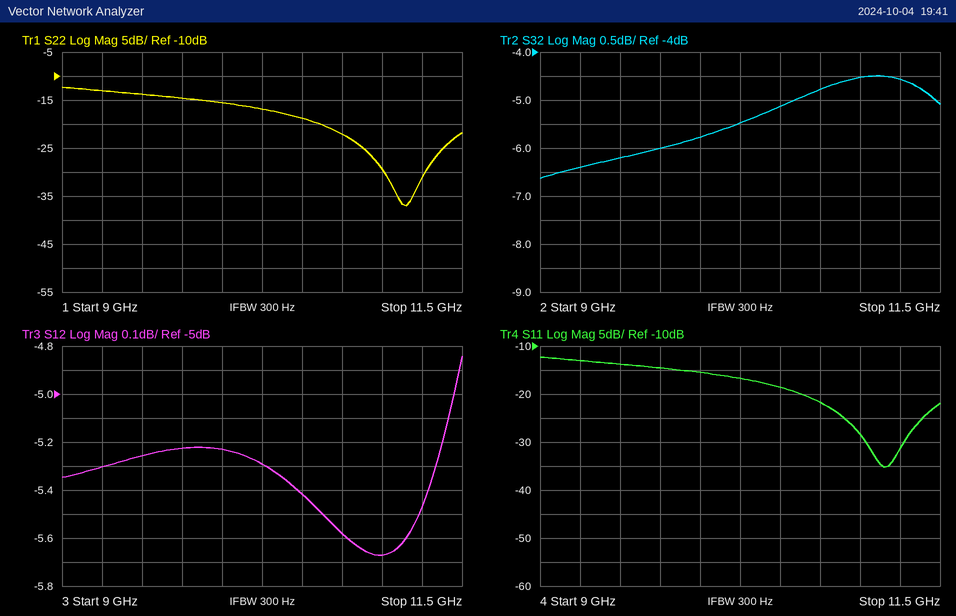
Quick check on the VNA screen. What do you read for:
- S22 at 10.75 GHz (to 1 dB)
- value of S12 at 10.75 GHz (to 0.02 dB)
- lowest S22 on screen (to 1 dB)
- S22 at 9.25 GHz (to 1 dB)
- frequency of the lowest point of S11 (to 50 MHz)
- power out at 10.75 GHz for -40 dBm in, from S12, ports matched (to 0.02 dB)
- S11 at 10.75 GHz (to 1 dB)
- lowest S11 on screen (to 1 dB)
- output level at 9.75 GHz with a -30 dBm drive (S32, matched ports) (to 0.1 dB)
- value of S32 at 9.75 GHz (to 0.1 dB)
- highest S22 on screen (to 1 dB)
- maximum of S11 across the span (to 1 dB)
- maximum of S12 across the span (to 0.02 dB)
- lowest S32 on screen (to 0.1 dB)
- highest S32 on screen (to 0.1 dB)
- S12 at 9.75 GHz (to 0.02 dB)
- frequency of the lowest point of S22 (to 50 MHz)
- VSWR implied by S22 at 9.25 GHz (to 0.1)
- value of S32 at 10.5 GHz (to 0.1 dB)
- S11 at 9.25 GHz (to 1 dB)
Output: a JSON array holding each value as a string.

["-22 dB", "-5.58 dB", "-37 dB", "-13 dB", "11.15 GHz", "-45.58 dBm", "-22 dB", "-35 dB", "-36.0 dBm", "-6.0 dB", "-12 dB", "-12 dB", "-4.84 dB", "-6.6 dB", "-4.5 dB", "-5.22 dB", "11.15 GHz", "1.6", "-5.1 dB", "-13 dB"]
